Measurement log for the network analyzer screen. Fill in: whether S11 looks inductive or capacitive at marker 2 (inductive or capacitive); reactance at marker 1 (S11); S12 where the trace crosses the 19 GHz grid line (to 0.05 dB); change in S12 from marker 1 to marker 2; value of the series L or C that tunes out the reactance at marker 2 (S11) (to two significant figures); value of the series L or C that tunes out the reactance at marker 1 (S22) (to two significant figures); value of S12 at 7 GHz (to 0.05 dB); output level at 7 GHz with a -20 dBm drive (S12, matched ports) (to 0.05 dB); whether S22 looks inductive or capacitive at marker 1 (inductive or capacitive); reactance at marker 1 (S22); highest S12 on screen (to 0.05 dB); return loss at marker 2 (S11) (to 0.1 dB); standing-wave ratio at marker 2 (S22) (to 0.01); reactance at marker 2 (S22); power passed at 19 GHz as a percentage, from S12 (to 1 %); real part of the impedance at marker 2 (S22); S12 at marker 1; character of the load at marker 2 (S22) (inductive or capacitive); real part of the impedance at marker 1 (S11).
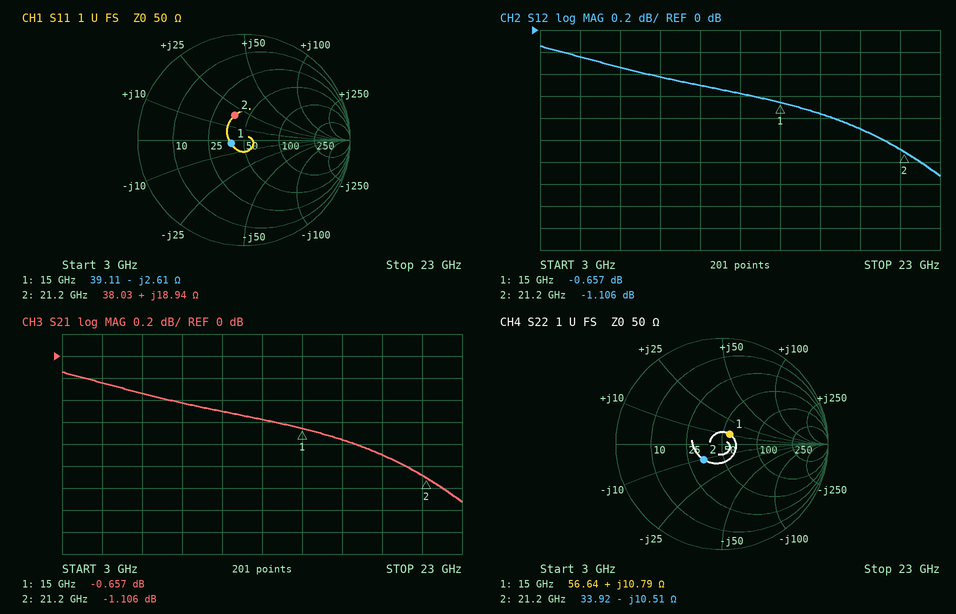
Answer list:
inductive
-2.61 Ω
-0.90 dB
-0.449 dB
400 fF
980 fF
-0.35 dB
-20.35 dBm
inductive
+10.79 Ω
-0.15 dB
12.1 dB
1.59
-10.51 Ω
81 %
33.92 Ω
-0.657 dB
capacitive
39.11 Ω
